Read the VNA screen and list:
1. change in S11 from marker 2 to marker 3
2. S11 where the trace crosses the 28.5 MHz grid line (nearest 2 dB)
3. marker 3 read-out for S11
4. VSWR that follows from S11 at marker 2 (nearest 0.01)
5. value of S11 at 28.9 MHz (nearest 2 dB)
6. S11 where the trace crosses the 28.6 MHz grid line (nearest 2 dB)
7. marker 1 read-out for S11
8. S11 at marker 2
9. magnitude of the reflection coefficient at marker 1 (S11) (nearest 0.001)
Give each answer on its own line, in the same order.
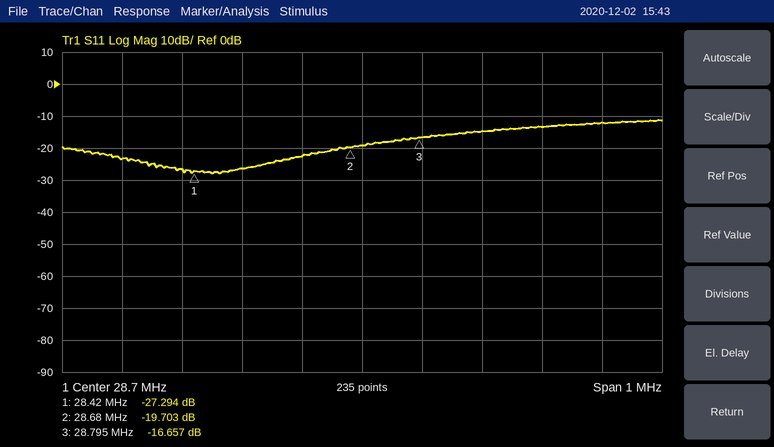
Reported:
3.046 dB
-26 dB
-16.657 dB
1.23
-14 dB
-22 dB
-27.294 dB
-19.703 dB
0.043
